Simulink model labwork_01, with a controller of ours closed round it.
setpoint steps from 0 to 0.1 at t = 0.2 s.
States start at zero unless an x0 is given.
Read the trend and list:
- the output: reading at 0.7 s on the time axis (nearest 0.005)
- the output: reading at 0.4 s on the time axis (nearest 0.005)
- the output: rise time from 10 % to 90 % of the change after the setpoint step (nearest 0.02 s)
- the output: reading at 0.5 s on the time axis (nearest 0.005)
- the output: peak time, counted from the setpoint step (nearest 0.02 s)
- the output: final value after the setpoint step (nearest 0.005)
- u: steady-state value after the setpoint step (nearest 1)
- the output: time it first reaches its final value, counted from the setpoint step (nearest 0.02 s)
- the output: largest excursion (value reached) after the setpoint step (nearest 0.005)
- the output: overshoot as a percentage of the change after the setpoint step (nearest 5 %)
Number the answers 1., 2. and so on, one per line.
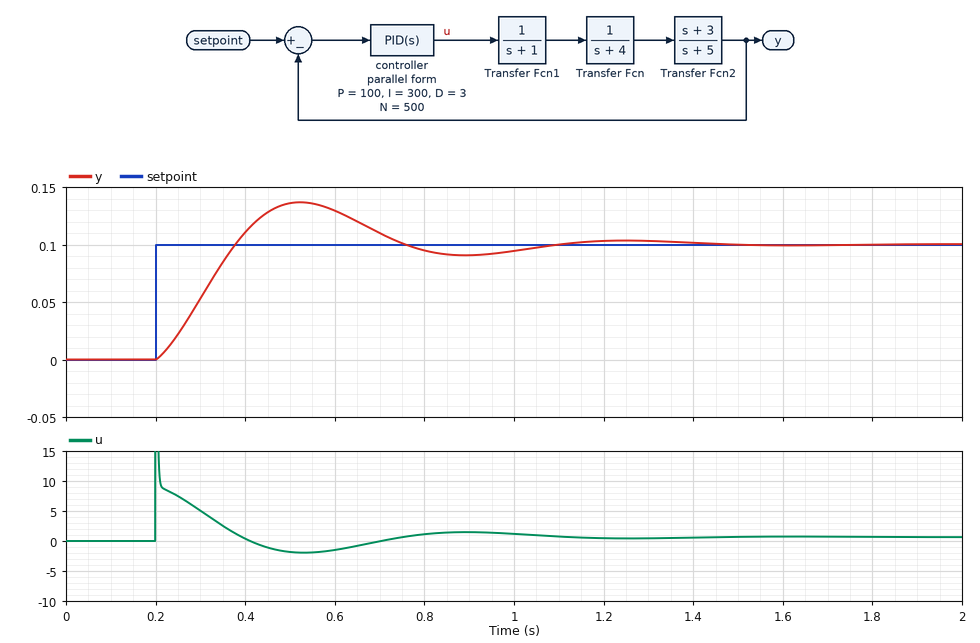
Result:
1. 0.110
2. 0.110
3. 0.14 s
4. 0.135
5. 0.32 s
6. 0.100
7. 1
8. 0.18 s
9. 0.135
10. 35 %
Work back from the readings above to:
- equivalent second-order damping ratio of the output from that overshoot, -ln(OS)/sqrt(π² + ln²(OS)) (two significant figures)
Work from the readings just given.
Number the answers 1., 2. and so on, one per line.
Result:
1. 0.32
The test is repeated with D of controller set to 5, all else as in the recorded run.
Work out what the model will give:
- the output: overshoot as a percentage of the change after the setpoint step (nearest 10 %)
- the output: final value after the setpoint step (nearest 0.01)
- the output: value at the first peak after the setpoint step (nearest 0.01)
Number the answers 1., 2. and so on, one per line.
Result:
1. 30 %
2. 0.10
3. 0.13
